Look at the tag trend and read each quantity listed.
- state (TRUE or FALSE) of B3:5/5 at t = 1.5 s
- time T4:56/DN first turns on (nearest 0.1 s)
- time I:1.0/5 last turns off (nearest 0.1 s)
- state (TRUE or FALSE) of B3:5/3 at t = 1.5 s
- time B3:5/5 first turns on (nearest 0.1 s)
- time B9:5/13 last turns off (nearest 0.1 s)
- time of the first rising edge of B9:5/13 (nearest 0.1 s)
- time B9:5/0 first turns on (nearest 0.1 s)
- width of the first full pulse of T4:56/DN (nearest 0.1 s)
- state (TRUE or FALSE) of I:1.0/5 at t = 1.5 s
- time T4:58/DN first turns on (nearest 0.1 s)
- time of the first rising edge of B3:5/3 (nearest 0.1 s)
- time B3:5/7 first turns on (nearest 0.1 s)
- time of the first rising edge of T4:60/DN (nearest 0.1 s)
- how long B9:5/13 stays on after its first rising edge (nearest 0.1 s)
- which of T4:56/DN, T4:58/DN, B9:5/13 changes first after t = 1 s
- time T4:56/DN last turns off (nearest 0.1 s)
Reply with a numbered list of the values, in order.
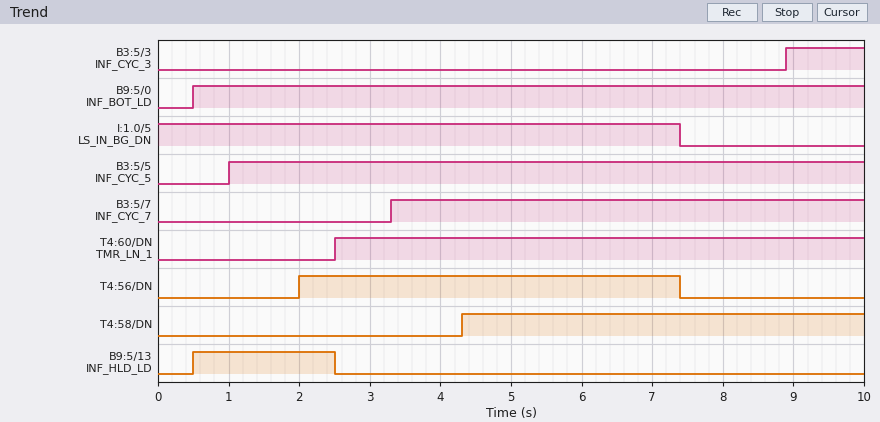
1. TRUE
2. 2.0 s
3. 7.4 s
4. FALSE
5. 1.0 s
6. 2.5 s
7. 0.5 s
8. 0.5 s
9. 5.4 s
10. TRUE
11. 4.3 s
12. 8.9 s
13. 3.3 s
14. 2.5 s
15. 2.0 s
16. T4:56/DN
17. 7.4 s
